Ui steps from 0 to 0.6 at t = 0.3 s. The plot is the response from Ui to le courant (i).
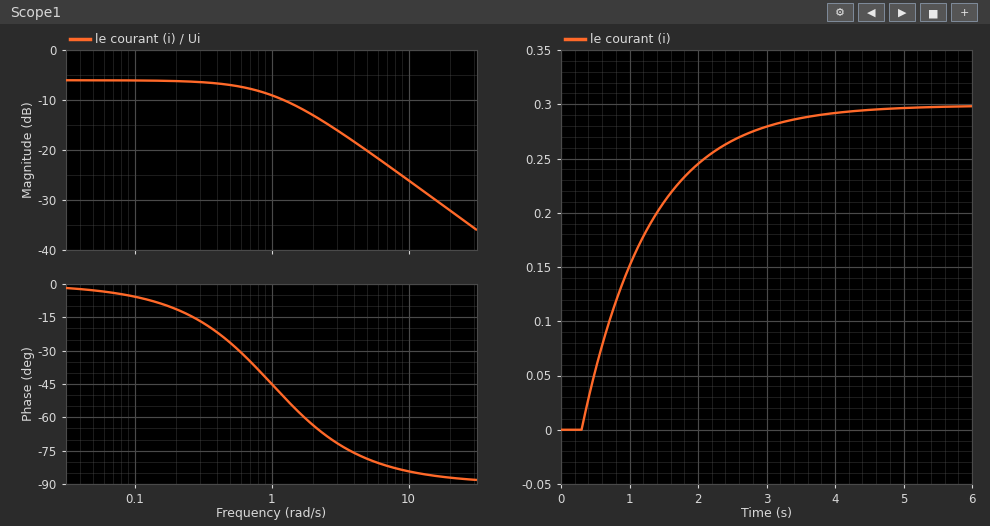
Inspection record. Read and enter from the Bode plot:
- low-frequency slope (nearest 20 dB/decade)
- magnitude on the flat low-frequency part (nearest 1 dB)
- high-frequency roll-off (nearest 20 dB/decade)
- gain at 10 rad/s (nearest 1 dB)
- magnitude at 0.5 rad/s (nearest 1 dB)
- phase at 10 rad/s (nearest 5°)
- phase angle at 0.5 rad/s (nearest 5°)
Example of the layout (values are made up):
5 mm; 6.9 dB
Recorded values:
0 dB/decade; -6 dB; -20 dB/decade; -26 dB; -7 dB; -85°; -25°
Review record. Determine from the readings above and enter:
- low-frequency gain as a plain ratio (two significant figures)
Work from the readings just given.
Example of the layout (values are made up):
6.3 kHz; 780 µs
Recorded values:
0.50
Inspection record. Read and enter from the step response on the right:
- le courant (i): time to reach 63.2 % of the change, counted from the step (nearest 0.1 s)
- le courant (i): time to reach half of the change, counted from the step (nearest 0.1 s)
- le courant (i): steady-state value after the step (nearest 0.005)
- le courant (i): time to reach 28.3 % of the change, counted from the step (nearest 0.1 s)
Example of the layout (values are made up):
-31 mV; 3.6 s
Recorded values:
1.0 s; 0.7 s; 0.300; 0.3 s
